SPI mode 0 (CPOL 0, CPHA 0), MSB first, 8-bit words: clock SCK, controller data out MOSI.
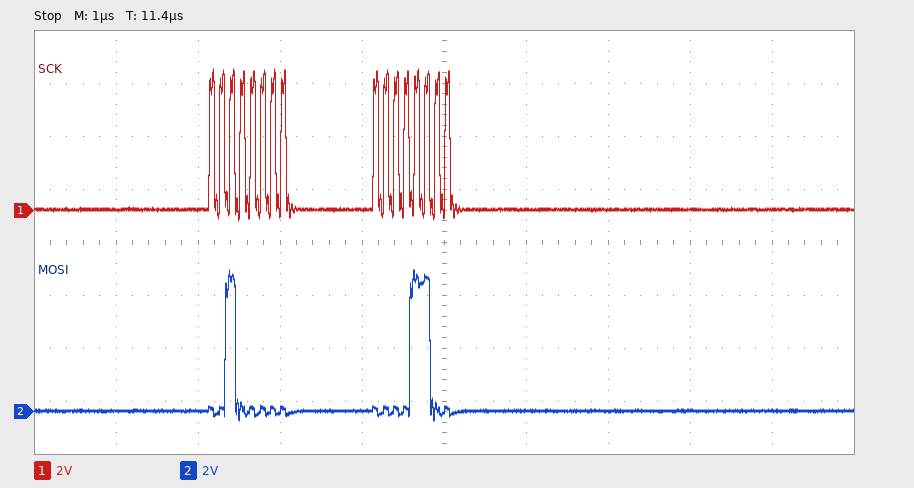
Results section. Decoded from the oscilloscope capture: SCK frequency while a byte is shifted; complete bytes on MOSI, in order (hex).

8 MHz
0x20 0x0C
